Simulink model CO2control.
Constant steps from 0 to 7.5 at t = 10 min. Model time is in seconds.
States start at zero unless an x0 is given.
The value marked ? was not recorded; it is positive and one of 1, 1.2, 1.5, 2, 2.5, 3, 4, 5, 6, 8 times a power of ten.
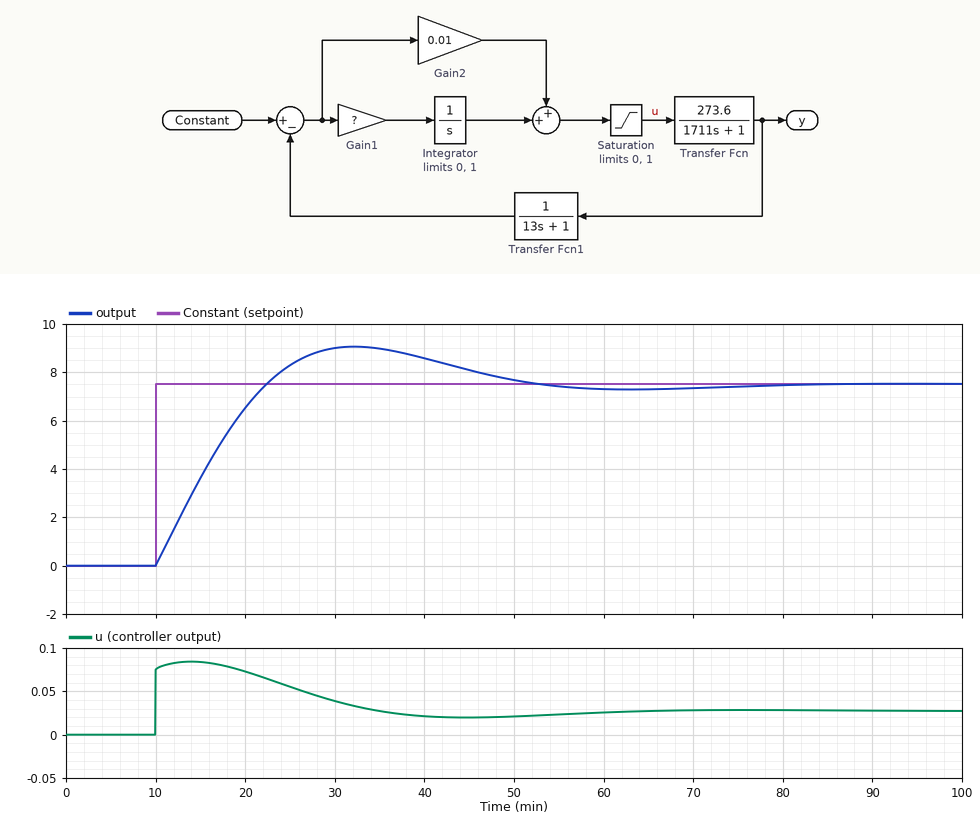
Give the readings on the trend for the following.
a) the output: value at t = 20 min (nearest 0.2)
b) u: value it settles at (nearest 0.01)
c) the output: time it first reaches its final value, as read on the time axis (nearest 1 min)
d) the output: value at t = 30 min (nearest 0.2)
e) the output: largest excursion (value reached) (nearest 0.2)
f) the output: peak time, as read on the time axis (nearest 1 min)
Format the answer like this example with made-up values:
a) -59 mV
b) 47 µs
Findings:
a) 6.6
b) 0.03
c) 22 min
d) 9.0
e) 9.0
f) 32 min
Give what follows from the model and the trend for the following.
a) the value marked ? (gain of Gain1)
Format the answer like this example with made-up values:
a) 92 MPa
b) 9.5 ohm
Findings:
a) 2.5e-05
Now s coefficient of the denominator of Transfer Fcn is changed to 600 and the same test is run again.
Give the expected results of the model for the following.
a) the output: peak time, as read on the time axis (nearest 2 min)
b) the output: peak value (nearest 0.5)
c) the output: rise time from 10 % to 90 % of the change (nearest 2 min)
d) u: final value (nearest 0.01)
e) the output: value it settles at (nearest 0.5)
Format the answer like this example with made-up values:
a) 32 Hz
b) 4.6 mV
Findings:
a) 24 min
b) 8.0
c) 6 min
d) 0.03
e) 7.5
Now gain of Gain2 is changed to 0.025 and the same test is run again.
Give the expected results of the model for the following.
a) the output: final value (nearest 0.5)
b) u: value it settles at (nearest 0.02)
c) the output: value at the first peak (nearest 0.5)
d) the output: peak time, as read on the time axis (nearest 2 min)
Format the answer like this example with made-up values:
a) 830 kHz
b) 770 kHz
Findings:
a) 7.5
b) 0.02
c) 8.0
d) 28 min
